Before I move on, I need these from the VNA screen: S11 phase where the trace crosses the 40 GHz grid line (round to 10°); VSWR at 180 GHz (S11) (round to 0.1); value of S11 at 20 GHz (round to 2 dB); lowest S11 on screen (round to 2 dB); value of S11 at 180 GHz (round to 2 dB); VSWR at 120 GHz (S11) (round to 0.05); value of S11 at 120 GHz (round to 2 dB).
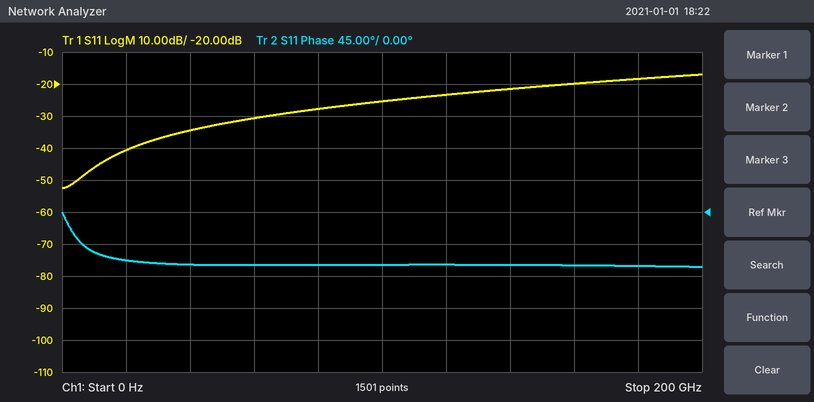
-70°
1.3
-40 dB
-52 dB
-18 dB
1.15
-24 dB
